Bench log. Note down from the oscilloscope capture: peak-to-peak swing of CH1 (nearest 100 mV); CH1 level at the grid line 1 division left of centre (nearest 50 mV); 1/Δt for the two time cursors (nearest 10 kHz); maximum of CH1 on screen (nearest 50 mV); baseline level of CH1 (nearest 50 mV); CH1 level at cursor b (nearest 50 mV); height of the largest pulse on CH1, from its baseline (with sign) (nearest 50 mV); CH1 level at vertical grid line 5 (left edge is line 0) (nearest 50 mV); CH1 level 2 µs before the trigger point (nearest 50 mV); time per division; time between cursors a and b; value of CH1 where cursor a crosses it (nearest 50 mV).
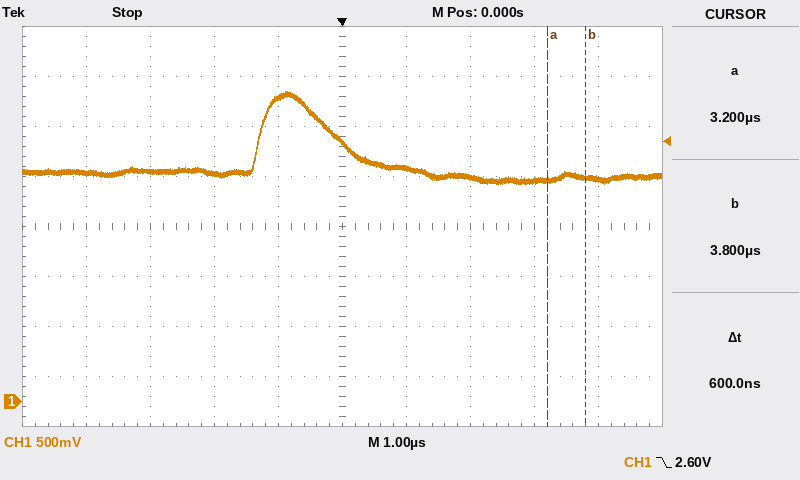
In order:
900 mV
3.05 V
1.67 MHz
3.10 V
2.30 V
2.25 V
+800 mV
2.60 V
2.30 V
1 µs
600 ns
2.20 V
